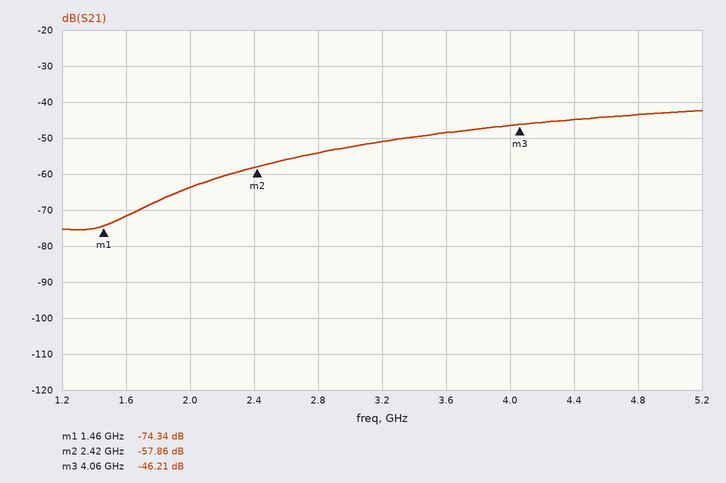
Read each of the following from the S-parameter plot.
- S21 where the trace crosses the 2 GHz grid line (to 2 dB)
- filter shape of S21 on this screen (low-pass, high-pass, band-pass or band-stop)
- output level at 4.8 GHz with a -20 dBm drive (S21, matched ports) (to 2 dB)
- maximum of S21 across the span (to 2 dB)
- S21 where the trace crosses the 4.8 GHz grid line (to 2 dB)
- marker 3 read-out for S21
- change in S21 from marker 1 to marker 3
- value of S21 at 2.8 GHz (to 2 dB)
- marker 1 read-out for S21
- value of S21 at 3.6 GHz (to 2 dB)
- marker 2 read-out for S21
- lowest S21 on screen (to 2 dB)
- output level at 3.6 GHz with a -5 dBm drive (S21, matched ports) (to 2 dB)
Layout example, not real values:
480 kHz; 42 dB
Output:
-64 dB; high-pass; -64 dBm; -42 dB; -44 dB; -46.21 dB; 28.13 dB; -54 dB; -74.34 dB; -48 dB; -57.86 dB; -76 dB; -54 dBm
